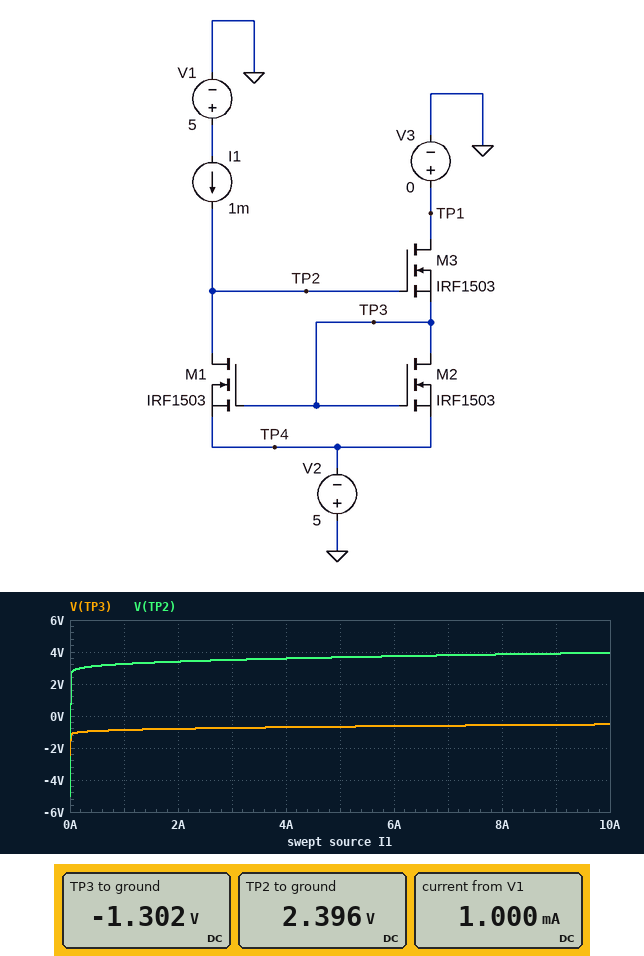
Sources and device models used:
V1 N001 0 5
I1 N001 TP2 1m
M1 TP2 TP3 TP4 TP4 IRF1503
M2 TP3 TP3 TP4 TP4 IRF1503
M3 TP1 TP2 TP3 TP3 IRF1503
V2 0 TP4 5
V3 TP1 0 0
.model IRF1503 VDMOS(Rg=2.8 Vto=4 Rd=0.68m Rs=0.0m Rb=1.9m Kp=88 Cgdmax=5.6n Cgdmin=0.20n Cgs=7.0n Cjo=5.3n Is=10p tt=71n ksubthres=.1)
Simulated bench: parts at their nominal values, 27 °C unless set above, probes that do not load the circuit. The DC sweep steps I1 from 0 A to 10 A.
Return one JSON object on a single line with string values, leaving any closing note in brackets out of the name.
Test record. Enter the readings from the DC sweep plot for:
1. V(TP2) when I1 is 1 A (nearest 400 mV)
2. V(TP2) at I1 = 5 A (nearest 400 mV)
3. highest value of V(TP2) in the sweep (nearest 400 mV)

{"V(TP2) when I1 is 1 A": "3.2 V", "V(TP2) at I1 = 5 A": "3.6 V", "highest value of V(TP2) in the sweep": "4.0 V"}
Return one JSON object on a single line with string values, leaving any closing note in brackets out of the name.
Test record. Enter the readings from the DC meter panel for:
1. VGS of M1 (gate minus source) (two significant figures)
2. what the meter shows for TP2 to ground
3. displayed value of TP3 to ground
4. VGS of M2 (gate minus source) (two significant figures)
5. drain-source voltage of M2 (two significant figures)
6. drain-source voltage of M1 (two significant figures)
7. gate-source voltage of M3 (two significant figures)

{"VGS of M1 (gate minus source)": "3.7 V", "what the meter shows for TP2 to ground": "2.396 V", "displayed value of TP3 to ground": "-1.302 V", "VGS of M2 (gate minus source)": "3.7 V", "drain-source voltage of M2": "3.7 V", "drain-source voltage of M1": "7.4 V", "gate-source voltage of M3": "3.7 V"}
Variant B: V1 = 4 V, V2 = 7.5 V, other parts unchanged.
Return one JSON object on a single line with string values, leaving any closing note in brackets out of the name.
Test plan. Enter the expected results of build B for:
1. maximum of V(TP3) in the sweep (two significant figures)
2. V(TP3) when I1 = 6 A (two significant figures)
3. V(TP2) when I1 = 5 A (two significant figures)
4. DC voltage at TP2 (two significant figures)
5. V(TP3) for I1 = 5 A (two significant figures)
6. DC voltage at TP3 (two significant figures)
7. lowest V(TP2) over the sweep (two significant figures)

{"maximum of V(TP3) in the sweep": "-3.0 V", "V(TP3) when I1 = 6 A": "-3.1 V", "V(TP2) when I1 = 5 A": "1.2 V", "DC voltage at TP2": "-100 mV", "V(TP3) for I1 = 5 A": "-3.2 V", "DC voltage at TP3": "-3.8 V", "lowest V(TP2) over the sweep": "-7.5 V"}
